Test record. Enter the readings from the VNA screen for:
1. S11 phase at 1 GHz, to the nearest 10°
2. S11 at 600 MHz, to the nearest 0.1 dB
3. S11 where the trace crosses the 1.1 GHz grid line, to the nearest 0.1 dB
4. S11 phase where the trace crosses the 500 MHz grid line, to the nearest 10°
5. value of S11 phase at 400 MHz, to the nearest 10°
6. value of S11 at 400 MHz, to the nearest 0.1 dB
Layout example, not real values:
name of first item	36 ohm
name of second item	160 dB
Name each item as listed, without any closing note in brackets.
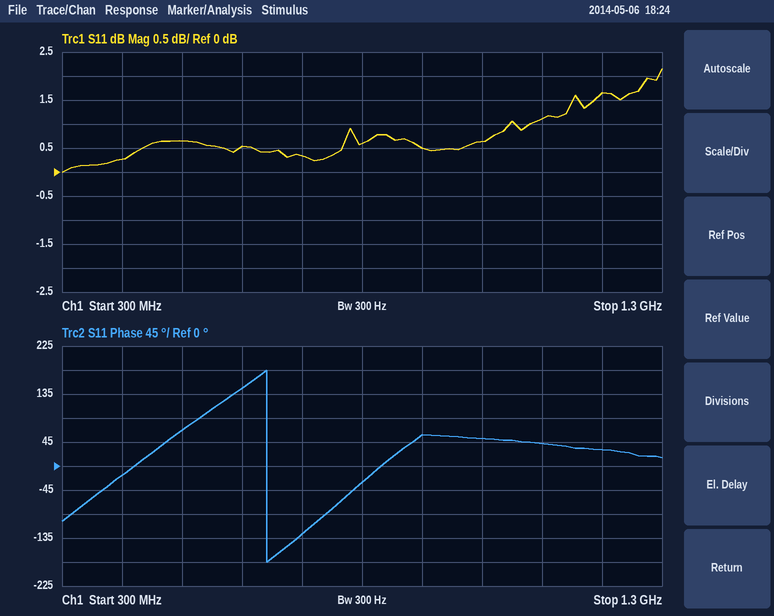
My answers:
S11 phase at 1 GHz, to the nearest 10°	50°
S11 at 600 MHz, to the nearest 0.1 dB	0.5 dB
S11 where the trace crosses the 1.1 GHz grid line, to the nearest 0.1 dB	1.1 dB
S11 phase where the trace crosses the 500 MHz grid line, to the nearest 10°	70°
value of S11 phase at 400 MHz, to the nearest 10°	-20°
value of S11 at 400 MHz, to the nearest 0.1 dB	0.3 dB
